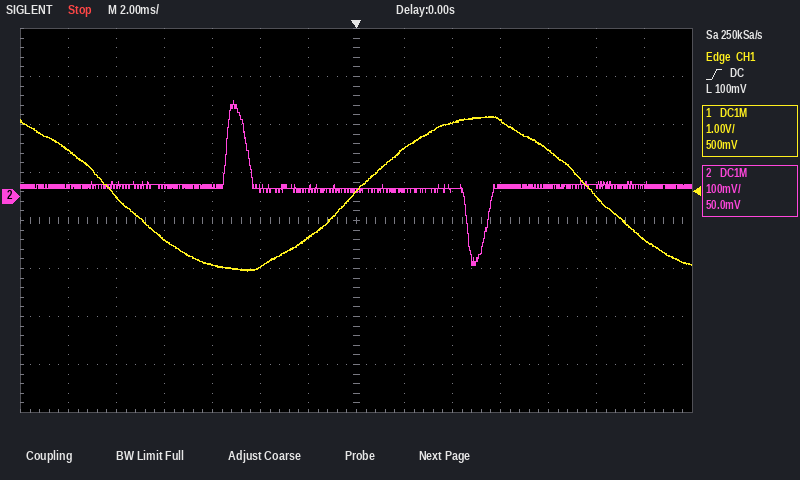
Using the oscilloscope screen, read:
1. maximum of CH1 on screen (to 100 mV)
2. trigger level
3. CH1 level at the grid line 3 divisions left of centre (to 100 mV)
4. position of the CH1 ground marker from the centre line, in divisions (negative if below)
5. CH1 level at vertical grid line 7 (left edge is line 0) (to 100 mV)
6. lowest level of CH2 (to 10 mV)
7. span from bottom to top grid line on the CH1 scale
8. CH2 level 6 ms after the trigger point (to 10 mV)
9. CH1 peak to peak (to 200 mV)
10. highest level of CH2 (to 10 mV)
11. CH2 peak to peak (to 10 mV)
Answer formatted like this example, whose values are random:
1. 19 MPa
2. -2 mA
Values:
1. 1.7 V
2. 100 mV
3. -1.4 V
4. +0.5 div
5. 100 mV
6. -140 mV
7. 8 V
8. 20 mV
9. 3.2 V
10. 200 mV
11. 340 mV
